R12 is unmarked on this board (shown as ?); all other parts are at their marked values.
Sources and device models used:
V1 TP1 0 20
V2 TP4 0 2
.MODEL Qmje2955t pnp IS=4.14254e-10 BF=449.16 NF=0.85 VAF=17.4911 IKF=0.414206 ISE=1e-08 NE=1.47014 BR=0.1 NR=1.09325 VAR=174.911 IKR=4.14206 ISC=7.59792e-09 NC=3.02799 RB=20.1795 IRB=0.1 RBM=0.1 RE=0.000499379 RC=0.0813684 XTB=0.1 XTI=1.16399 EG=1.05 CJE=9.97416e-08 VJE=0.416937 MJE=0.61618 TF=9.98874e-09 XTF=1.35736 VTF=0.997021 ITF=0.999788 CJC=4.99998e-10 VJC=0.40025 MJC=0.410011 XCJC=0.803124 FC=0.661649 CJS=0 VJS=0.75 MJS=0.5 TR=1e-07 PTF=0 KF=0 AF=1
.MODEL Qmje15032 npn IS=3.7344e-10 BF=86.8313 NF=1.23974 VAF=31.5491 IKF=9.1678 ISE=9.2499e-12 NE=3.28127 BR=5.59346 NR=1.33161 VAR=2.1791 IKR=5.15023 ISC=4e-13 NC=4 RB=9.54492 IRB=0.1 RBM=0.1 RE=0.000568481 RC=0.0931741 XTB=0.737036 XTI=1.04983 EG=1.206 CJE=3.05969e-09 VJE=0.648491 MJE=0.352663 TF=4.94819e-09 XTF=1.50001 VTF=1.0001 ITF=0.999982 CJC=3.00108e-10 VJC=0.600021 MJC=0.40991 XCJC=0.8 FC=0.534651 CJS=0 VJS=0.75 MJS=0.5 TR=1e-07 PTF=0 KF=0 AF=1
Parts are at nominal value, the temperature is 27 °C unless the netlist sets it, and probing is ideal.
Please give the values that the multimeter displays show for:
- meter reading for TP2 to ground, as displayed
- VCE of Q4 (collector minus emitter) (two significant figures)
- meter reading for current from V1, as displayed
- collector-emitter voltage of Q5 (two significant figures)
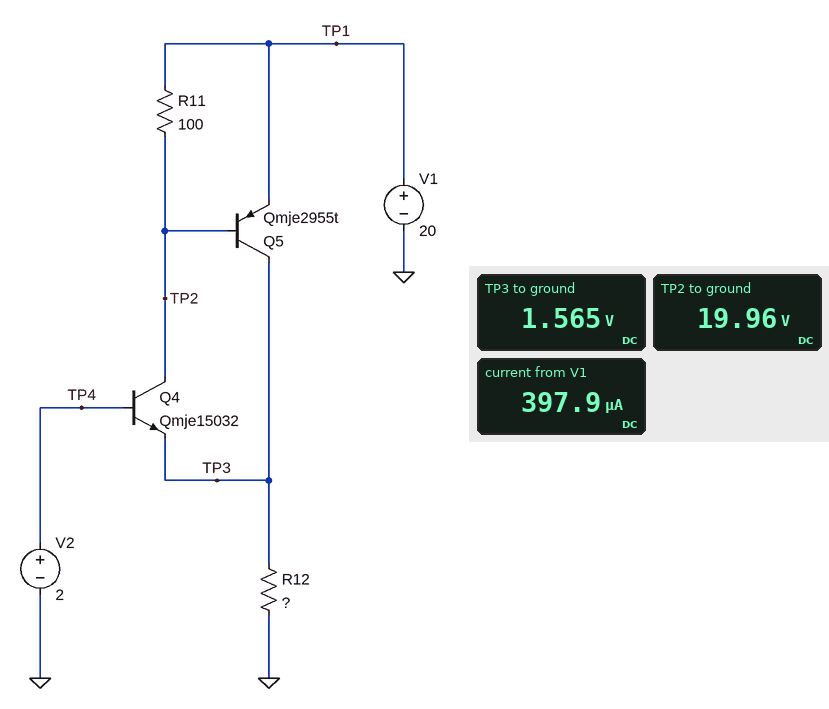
19.96 V
18 V
397.9 µA
-18 V
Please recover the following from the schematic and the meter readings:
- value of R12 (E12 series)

3.9 kΩ
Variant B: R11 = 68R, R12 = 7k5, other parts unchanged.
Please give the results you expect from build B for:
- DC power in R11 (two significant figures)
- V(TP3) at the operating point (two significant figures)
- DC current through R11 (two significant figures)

3.0 µW
1.6 V
210 µA
